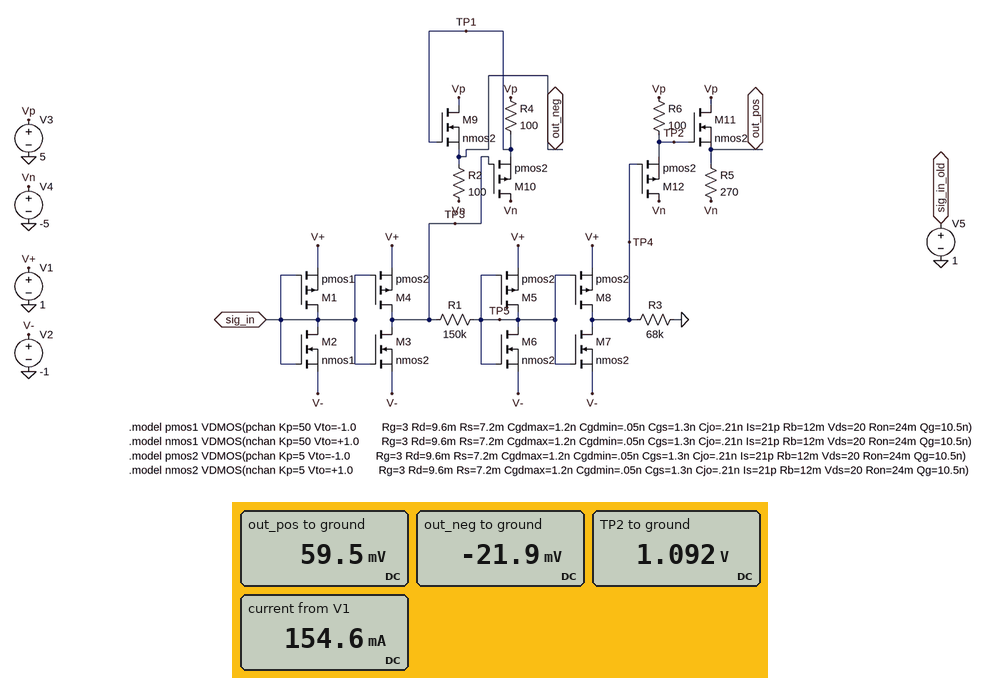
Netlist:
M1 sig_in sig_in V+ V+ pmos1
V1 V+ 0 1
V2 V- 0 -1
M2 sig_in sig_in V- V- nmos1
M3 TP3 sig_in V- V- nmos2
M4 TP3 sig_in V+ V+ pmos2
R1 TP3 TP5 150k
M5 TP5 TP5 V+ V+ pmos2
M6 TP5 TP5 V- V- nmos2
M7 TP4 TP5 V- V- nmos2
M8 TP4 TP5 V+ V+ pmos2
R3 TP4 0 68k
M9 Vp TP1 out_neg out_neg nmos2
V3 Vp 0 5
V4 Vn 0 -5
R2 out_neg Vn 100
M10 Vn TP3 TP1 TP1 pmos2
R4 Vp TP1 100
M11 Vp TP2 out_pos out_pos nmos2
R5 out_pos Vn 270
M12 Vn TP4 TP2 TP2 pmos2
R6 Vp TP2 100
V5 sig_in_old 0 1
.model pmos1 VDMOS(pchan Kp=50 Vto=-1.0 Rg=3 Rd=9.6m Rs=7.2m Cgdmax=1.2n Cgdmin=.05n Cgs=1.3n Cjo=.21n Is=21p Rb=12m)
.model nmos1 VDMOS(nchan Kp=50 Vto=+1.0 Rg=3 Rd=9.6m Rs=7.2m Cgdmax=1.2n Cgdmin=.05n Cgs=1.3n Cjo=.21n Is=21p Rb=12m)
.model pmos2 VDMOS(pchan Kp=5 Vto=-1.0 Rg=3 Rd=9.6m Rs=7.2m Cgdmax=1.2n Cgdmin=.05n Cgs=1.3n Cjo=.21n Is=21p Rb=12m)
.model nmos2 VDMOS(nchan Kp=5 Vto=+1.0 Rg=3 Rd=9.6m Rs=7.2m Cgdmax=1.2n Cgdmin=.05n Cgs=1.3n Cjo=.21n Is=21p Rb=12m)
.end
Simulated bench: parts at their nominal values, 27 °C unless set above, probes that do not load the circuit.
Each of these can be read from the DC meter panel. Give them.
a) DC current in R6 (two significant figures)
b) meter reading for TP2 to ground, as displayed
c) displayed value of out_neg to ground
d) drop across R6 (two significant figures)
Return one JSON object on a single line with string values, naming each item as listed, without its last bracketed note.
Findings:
{"DC current in R6": "39 mA", "meter reading for TP2 to ground, as displayed": "1.092 V", "displayed value of out_neg to ground": "-21.9 mV", "drop across R6": "3.9 V"}
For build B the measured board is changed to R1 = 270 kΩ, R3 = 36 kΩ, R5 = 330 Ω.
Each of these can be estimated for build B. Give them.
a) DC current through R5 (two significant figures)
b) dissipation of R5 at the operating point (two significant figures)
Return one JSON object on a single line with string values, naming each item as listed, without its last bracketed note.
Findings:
{"DC current through R5": "15 mA", "dissipation of R5 at the operating point": "78 mW"}
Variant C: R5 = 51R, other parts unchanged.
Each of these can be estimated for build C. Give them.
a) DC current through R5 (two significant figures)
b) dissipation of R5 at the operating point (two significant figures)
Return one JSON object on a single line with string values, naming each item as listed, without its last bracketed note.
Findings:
{"DC current through R5": "96 mA", "dissipation of R5 at the operating point": "470 mW"}
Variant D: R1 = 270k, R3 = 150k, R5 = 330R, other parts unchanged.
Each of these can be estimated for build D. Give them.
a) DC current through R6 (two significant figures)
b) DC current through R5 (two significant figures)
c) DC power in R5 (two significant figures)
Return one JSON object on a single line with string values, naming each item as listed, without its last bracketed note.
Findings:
{"DC current through R6": "39 mA", "DC current through R5": "15 mA", "DC power in R5": "78 mW"}
